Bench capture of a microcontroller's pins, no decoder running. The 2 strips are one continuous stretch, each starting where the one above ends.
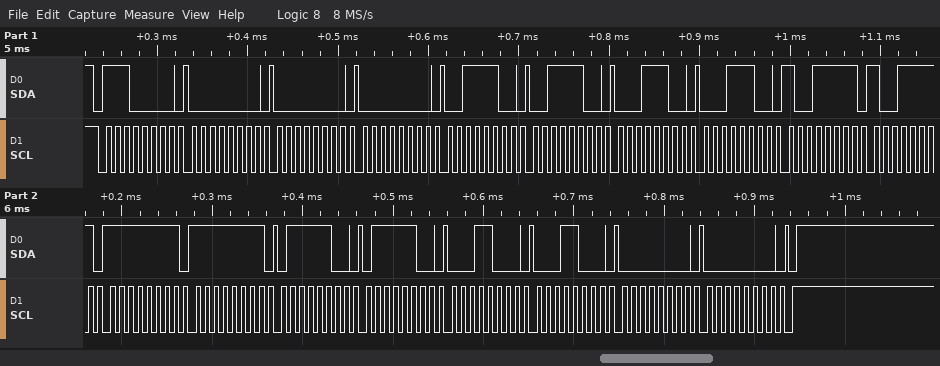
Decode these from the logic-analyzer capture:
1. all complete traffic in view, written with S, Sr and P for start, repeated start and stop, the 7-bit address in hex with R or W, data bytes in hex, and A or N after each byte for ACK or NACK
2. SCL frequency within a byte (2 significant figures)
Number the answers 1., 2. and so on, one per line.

1. S 70W A 00 A 00 A 00 A 3C A 3C A 1C A 1C A 9F A 9F A FF A FF A 7C A 7C A 18 A 18 A 00 A 00 A P
2. 100 kHz
